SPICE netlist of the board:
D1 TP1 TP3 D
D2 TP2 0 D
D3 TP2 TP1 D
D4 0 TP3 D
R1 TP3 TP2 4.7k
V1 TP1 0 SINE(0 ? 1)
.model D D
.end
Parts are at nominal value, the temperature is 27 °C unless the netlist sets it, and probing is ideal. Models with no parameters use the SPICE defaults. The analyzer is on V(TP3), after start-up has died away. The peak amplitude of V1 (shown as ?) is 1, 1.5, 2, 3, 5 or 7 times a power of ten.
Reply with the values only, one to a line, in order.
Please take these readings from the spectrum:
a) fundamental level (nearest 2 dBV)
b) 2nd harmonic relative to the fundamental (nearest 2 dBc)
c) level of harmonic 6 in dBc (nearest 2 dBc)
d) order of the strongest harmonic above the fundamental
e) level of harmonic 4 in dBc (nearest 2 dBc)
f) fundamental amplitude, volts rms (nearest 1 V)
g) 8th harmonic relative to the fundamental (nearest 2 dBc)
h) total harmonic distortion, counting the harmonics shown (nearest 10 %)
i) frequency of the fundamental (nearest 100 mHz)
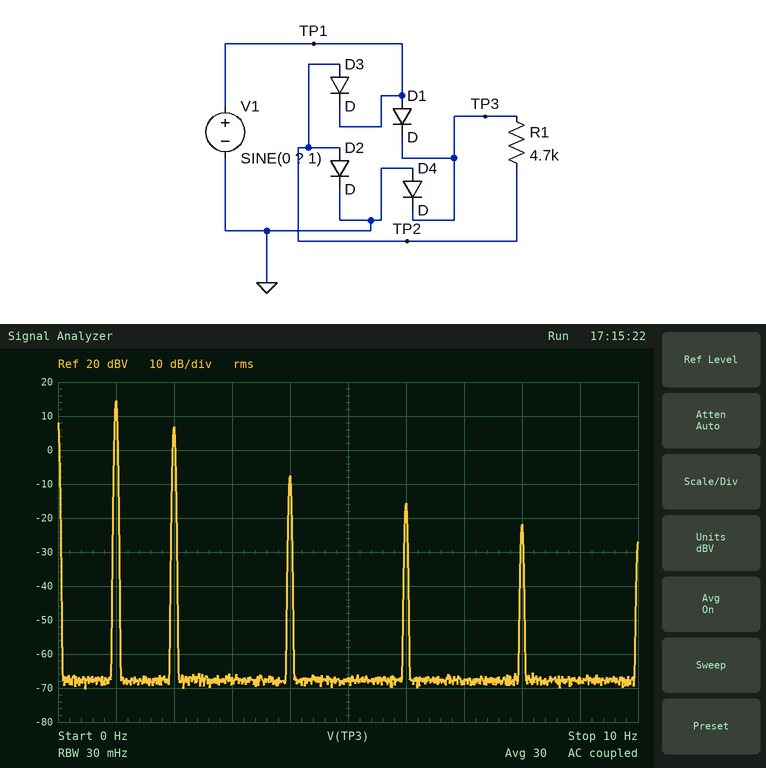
14 dBV
-8 dBc
-30 dBc
2
-22 dBc
5 V
-36 dBc
40 %
1.0 Hz
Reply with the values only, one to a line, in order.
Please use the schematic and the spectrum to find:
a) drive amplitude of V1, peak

15 V
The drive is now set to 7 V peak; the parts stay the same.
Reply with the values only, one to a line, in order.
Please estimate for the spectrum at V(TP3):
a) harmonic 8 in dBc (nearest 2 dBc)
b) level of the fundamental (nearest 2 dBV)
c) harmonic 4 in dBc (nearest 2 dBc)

-48 dBc
8 dBV
-24 dBc
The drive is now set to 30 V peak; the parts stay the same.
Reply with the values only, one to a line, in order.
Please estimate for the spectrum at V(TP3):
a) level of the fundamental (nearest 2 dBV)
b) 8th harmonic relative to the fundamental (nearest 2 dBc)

20 dBV
-34 dBc
